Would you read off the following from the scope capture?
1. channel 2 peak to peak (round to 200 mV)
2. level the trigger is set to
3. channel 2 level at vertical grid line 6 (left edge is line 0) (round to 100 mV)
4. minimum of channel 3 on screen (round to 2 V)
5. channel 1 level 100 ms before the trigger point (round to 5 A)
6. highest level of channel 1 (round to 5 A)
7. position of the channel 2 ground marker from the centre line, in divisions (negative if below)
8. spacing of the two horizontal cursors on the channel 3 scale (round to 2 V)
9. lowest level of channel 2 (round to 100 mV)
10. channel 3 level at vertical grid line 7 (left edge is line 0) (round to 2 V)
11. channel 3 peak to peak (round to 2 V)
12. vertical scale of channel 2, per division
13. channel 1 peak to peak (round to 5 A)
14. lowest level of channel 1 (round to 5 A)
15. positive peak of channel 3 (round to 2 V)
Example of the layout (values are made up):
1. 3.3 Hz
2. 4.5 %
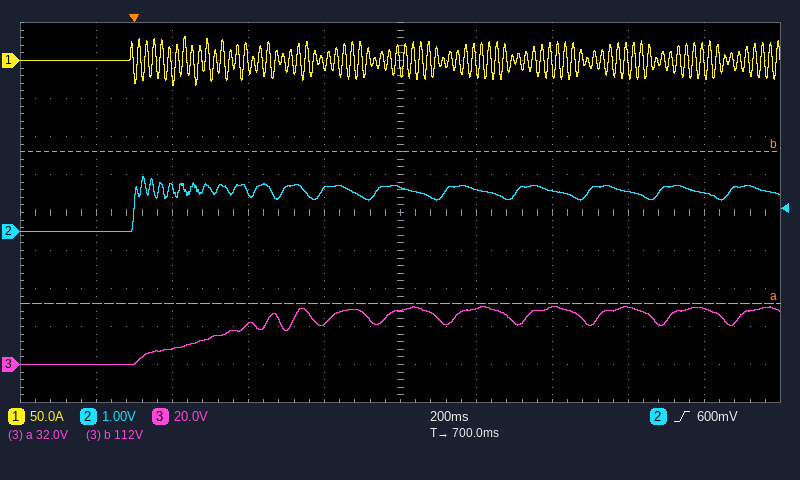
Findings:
1. 1.4 V
2. 600 mV
3. 1.1 V
4. 0 V
5. 0 A
6. 30 A
7. -0.5 div
8. 80 V
9. 0.0 V
10. 30 V
11. 30 V
12. 1 V
13. 65 A
14. -35 A
15. 30 V
